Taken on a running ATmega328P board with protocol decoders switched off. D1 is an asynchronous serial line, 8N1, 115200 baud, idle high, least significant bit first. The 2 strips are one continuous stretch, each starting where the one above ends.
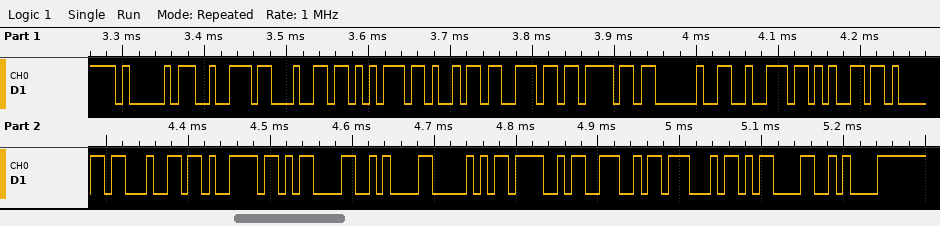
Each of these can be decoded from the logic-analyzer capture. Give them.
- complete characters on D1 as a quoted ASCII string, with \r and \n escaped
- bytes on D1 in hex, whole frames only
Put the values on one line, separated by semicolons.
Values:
"Arduino ready\r\nPONG\r\n"; 41 72 64 75 69 6E 6F 20 72 65 61 64 79 0D 0A 50 4F 4E 47 0D 0A
